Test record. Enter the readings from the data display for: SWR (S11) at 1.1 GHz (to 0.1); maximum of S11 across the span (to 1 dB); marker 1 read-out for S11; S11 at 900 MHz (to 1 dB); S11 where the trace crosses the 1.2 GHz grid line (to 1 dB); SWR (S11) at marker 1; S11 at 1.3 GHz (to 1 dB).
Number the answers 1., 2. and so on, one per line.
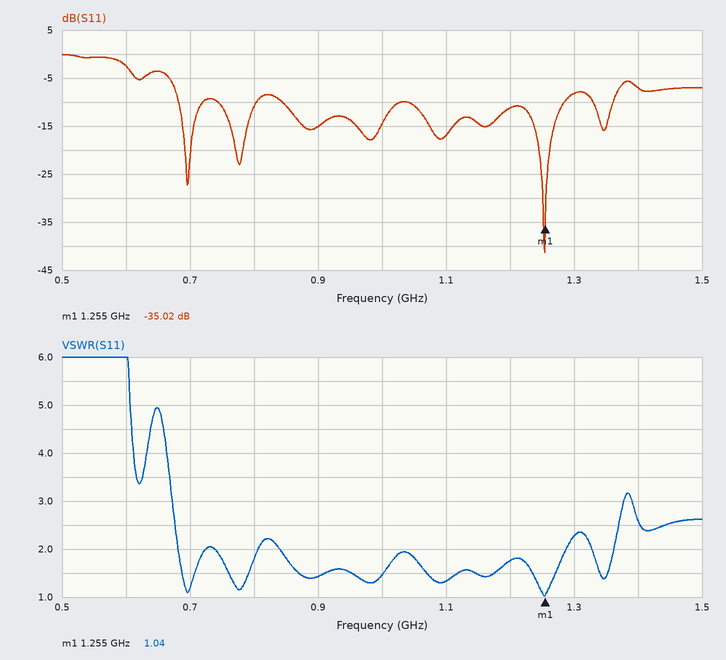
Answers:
1. 1.3
2. 0 dB
3. -35.02 dB
4. -15 dB
5. -11 dB
6. 1.04
7. -8 dB
